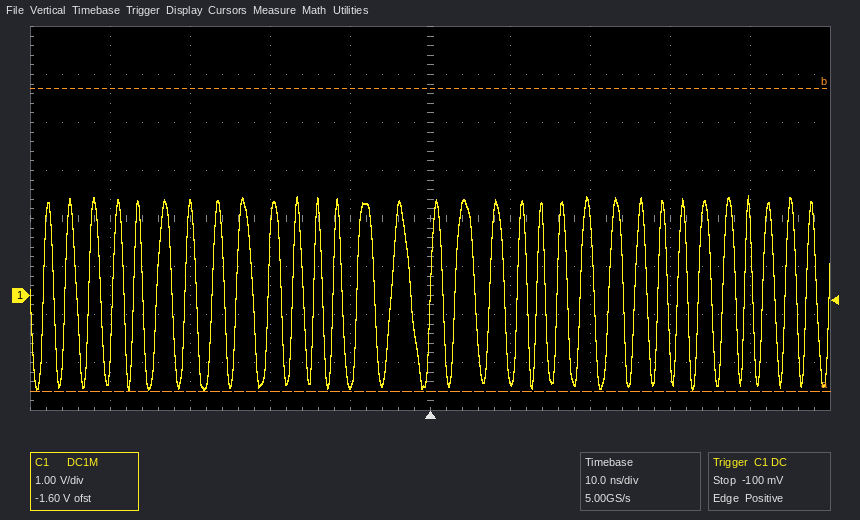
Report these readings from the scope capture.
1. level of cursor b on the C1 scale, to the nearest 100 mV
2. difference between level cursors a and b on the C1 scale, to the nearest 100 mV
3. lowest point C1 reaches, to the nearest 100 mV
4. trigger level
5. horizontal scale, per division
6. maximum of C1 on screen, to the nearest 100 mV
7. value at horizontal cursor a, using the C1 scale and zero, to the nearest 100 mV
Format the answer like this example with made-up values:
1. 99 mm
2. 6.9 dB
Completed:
1. 4.3 V
2. 6.3 V
3. -2.0 V
4. -100 mV
5. 10 ns
6. 2.1 V
7. -2.0 V
